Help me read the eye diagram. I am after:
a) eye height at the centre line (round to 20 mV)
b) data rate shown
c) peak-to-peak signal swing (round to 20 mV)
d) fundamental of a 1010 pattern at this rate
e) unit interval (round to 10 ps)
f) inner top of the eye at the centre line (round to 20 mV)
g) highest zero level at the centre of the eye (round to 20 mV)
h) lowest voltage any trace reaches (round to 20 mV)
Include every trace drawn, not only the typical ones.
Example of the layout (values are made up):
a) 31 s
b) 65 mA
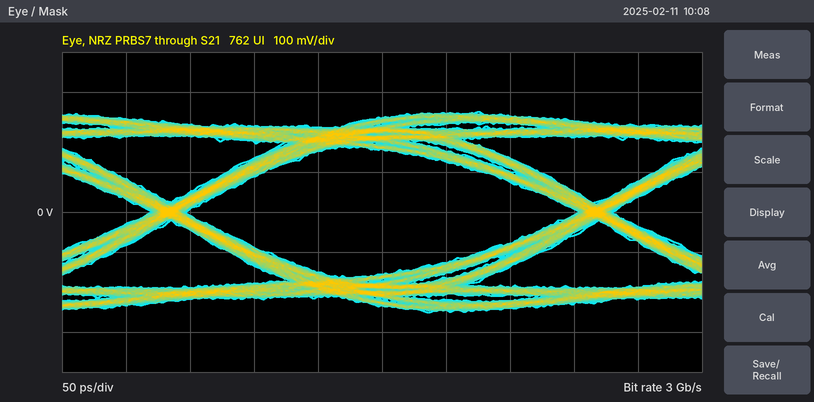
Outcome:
a) 320 mV
b) 3 Gb/s
c) 500 mV
d) 1.5 GHz
e) 330 ps
f) 160 mV
g) -160 mV
h) -260 mV
